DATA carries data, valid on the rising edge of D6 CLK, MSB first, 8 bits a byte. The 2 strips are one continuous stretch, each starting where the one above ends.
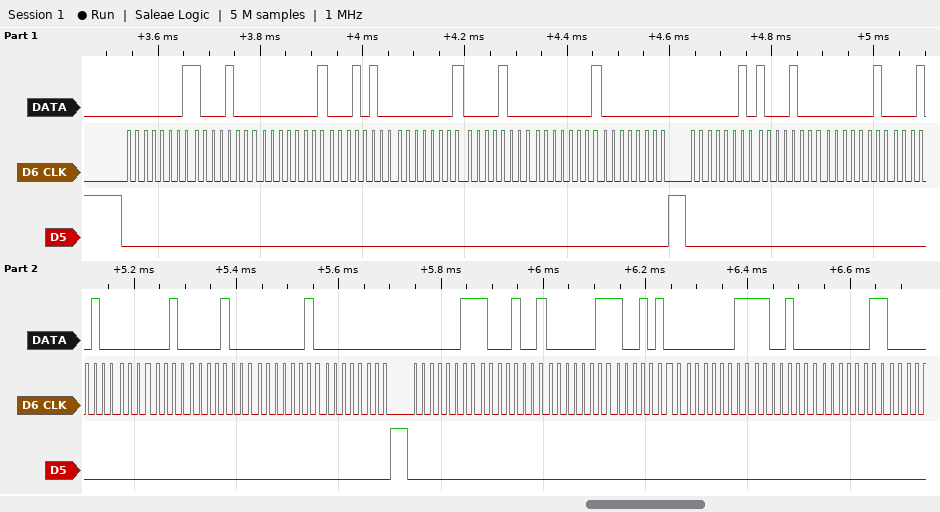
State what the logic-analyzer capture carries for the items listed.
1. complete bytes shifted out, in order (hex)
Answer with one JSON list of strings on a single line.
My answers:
["01 88 01 14 01 08 01 00 02 88 02 14 02 08 02 00 03 89 03 94 03 C8 03"]
